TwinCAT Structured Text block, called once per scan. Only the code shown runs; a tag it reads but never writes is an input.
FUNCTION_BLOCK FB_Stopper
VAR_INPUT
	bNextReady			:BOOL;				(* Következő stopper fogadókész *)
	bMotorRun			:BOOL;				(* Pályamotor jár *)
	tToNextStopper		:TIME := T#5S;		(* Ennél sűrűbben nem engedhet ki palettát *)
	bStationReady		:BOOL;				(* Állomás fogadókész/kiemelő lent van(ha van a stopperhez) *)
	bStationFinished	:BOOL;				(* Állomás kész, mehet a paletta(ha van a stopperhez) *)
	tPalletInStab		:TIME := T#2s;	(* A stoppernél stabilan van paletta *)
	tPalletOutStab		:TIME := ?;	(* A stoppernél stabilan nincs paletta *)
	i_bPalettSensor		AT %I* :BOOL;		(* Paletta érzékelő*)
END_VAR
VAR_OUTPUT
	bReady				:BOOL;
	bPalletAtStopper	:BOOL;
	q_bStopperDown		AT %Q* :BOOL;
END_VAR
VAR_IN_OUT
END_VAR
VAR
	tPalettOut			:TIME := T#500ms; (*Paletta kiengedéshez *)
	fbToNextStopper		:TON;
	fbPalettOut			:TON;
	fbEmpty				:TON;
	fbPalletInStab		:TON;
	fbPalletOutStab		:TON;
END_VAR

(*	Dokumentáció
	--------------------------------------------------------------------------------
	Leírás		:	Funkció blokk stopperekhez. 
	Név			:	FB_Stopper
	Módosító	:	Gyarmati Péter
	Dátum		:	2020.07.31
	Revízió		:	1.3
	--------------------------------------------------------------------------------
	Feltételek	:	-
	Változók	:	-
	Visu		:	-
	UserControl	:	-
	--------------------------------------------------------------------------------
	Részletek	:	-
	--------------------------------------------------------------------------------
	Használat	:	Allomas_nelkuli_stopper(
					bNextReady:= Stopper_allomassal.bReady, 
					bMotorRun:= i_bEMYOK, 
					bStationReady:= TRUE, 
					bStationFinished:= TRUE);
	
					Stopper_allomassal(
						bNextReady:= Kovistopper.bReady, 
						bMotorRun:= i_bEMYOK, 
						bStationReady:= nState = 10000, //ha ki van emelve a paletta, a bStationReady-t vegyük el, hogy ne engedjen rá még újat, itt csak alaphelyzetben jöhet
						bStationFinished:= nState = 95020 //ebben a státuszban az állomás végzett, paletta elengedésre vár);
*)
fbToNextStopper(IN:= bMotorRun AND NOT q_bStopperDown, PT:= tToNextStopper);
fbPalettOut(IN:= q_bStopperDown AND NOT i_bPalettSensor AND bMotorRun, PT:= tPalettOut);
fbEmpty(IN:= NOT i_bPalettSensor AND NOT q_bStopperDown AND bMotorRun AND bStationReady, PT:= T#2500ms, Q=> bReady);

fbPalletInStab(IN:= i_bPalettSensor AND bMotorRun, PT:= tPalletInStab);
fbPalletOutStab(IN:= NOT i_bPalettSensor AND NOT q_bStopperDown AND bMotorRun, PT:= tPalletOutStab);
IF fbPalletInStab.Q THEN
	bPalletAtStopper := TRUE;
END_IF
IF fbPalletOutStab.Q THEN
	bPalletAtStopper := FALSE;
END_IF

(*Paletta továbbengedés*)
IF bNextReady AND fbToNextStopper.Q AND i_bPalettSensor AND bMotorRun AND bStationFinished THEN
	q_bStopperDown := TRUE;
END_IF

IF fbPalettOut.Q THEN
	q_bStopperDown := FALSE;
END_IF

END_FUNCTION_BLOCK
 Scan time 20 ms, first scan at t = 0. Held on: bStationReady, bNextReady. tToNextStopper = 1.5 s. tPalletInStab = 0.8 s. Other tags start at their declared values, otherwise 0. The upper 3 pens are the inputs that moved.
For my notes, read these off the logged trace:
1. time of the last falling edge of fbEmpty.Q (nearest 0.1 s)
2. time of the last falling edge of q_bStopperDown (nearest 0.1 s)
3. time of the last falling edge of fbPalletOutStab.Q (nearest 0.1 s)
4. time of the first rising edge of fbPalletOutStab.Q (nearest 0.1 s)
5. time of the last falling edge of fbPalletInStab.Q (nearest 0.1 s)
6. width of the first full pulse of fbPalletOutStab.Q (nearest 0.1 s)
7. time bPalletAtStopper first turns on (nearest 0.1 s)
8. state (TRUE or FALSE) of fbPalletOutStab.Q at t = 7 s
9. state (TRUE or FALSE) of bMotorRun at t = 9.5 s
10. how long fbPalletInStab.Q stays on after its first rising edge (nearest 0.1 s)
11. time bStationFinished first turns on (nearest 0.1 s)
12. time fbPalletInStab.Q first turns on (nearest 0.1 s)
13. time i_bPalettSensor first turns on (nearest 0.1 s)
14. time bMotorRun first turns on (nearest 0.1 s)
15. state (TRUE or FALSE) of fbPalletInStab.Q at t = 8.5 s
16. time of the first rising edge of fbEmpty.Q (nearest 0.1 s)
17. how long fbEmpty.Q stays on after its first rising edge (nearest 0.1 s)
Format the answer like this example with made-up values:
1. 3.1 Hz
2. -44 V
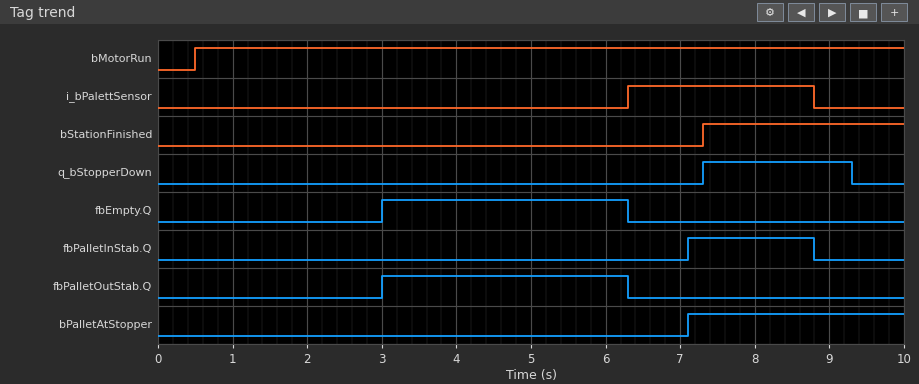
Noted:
1. 6.3 s
2. 9.3 s
3. 6.3 s
4. 3.0 s
5. 8.8 s
6. 3.3 s
7. 7.1 s
8. FALSE
9. TRUE
10. 1.7 s
11. 7.3 s
12. 7.1 s
13. 6.3 s
14. 0.5 s
15. TRUE
16. 3.0 s
17. 3.3 s
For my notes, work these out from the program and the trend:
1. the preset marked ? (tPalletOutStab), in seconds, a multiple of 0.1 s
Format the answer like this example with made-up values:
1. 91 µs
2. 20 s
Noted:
1. 2.5 s
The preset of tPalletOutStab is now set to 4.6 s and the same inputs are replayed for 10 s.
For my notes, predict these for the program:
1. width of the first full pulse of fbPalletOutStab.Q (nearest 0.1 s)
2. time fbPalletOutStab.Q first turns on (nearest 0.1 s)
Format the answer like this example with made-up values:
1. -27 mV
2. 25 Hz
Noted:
1. 1.2 s
2. 5.1 s
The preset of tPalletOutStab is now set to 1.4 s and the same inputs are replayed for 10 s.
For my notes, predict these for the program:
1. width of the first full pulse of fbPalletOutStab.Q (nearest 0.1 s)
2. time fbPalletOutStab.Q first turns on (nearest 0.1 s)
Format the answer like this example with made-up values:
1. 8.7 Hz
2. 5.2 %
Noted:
1. 4.4 s
2. 1.9 s
